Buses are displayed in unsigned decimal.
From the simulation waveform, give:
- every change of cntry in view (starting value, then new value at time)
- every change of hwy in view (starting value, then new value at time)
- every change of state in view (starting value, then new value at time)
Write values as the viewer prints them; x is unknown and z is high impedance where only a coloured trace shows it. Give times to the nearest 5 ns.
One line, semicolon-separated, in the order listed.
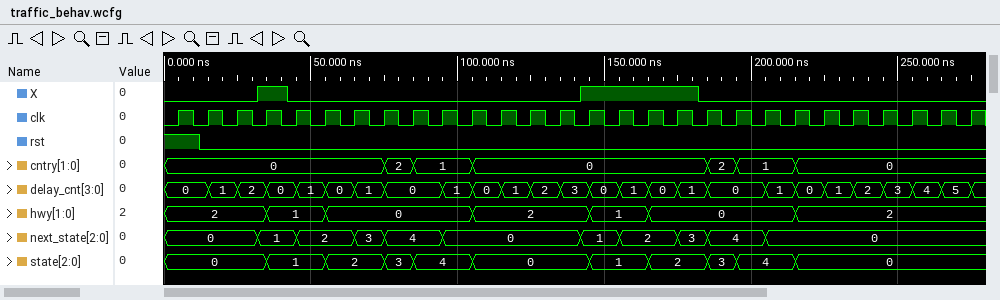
0, 2 at 75 ns, 1 at 85 ns, 0 at 105 ns, 2 at 185 ns, 1 at 195 ns, 0 at 215 ns; 2, 1 at 35 ns, 0 at 55 ns, 2 at 105 ns, 1 at 145 ns, 0 at 165 ns, 2 at 215 ns; 0, 1 at 35 ns, 2 at 55 ns, 3 at 75 ns, 4 at 85 ns, 0 at 105 ns, 1 at 145 ns, 2 at 165 ns, 3 at 185 ns, 4 at 195 ns, 0 at 215 ns
